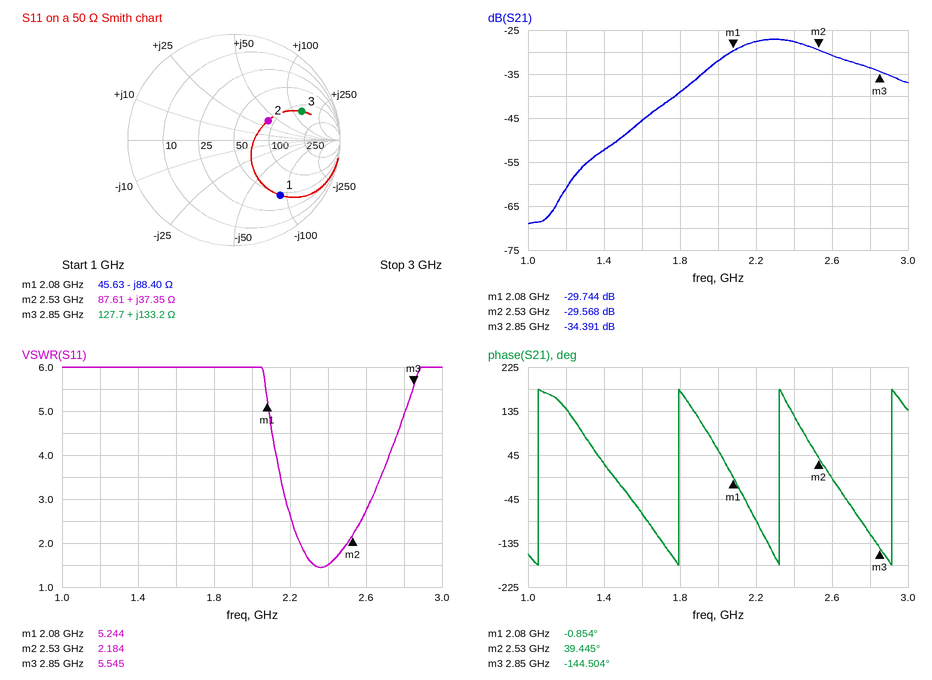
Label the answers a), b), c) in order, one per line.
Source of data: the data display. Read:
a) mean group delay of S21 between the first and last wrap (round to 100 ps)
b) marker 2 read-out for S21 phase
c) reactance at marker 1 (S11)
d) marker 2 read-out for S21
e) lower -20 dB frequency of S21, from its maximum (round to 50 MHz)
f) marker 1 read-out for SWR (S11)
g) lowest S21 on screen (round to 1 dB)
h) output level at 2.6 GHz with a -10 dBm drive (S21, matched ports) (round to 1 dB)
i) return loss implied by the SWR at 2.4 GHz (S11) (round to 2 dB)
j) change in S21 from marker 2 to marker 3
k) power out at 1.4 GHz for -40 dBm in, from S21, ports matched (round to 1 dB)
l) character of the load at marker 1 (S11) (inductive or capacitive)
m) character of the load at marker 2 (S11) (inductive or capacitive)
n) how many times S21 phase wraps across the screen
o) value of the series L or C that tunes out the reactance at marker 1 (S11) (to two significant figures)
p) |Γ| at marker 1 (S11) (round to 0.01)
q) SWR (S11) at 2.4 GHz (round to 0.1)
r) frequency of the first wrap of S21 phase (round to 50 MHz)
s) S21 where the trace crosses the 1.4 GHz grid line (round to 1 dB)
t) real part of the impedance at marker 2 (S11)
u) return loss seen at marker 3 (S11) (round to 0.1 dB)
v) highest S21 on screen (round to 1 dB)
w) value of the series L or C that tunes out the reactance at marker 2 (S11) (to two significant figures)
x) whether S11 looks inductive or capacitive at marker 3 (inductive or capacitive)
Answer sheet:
a) 1.6 ns
b) 39.445°
c) -88.40 Ω
d) -29.568 dB
e) 1.55 GHz
f) 5.244
g) -69 dB
h) -41 dBm
i) 14 dB
j) -4.823 dB
k) -92 dBm
l) capacitive
m) inductive
n) 4
o) 6.8 nH
p) 0.68
q) 1.5
r) 1.05 GHz
s) -52 dB
t) 87.61 Ω
u) 3.2 dB
v) -27 dB
w) 1.7 pF
x) inductive
